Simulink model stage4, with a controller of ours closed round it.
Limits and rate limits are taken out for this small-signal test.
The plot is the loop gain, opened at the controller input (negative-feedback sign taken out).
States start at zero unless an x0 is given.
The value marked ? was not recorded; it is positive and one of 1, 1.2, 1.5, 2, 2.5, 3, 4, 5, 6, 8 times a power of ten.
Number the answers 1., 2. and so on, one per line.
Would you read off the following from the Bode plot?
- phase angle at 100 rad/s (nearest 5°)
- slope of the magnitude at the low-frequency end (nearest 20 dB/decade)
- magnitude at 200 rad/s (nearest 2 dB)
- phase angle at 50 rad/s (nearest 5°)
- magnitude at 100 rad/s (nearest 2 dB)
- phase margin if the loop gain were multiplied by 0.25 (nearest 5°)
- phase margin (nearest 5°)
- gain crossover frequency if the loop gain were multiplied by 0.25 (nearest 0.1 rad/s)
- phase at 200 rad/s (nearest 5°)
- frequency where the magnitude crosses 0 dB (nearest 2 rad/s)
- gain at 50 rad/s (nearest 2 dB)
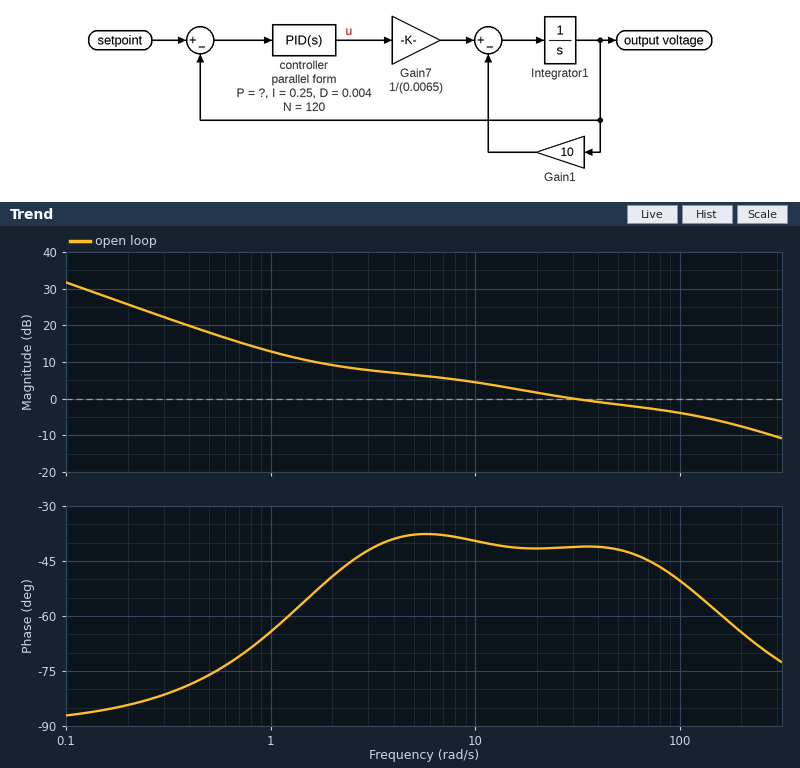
1. -50°
2. -20 dB/decade
3. -8 dB
4. -40°
5. -4 dB
6. 120°
7. 140°
8. 1.1 rad/s
9. -65°
10. 30 rad/s
11. -2 dB
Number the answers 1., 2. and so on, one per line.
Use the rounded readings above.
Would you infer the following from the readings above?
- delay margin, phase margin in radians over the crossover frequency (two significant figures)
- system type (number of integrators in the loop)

1. 0.081 s
2. 1
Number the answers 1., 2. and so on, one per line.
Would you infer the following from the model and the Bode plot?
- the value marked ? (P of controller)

1. 0.15
